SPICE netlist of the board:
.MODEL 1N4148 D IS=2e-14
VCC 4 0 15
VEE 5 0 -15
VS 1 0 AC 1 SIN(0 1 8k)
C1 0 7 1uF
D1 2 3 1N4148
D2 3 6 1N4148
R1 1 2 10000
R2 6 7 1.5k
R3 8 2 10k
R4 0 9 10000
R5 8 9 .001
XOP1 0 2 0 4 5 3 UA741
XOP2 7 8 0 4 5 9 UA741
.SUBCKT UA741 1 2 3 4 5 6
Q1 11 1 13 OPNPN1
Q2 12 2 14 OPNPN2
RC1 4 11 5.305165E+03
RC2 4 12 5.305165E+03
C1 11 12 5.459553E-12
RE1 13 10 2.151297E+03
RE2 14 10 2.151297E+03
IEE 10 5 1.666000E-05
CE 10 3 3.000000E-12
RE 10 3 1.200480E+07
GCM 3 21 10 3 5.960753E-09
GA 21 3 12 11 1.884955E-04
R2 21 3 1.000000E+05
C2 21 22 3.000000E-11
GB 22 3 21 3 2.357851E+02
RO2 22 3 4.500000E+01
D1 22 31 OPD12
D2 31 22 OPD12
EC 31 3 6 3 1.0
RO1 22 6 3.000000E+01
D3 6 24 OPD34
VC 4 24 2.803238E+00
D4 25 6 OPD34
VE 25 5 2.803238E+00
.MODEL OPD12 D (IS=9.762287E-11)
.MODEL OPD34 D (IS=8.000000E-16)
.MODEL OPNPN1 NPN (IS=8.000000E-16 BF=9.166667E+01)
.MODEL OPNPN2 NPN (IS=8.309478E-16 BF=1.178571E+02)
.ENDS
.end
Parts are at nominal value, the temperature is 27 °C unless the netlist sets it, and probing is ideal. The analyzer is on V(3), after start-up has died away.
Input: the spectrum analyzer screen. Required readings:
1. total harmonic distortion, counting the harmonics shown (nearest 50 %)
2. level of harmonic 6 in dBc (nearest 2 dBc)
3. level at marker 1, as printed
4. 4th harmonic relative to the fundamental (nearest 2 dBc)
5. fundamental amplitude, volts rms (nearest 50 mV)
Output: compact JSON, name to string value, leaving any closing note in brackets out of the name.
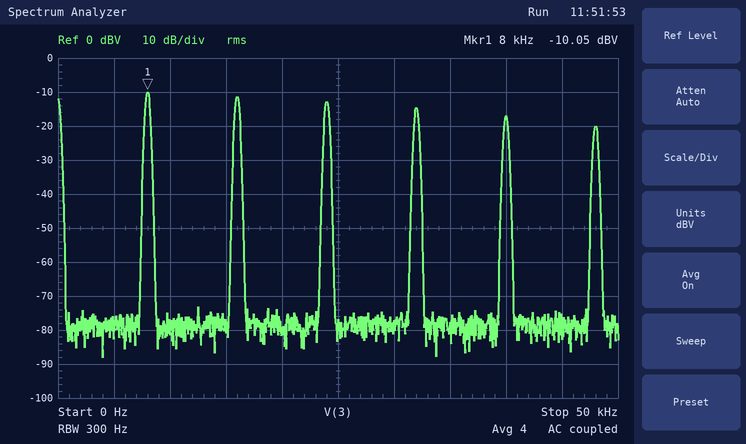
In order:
{"total harmonic distortion, counting the harmonics shown": "150 %", "level of harmonic 6 in dBc": "-10 dBc", "level at marker 1, as printed": "-10.05 dBV", "4th harmonic relative to the fundamental": "-4 dBc", "fundamental amplitude, volts rms": "300 mV"}
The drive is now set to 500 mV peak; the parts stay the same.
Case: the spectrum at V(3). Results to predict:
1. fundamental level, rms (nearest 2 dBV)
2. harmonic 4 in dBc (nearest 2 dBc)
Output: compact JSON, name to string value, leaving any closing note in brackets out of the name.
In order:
{"fundamental level, rms": "-12 dBV", "harmonic 4 in dBc": "-6 dBc"}
